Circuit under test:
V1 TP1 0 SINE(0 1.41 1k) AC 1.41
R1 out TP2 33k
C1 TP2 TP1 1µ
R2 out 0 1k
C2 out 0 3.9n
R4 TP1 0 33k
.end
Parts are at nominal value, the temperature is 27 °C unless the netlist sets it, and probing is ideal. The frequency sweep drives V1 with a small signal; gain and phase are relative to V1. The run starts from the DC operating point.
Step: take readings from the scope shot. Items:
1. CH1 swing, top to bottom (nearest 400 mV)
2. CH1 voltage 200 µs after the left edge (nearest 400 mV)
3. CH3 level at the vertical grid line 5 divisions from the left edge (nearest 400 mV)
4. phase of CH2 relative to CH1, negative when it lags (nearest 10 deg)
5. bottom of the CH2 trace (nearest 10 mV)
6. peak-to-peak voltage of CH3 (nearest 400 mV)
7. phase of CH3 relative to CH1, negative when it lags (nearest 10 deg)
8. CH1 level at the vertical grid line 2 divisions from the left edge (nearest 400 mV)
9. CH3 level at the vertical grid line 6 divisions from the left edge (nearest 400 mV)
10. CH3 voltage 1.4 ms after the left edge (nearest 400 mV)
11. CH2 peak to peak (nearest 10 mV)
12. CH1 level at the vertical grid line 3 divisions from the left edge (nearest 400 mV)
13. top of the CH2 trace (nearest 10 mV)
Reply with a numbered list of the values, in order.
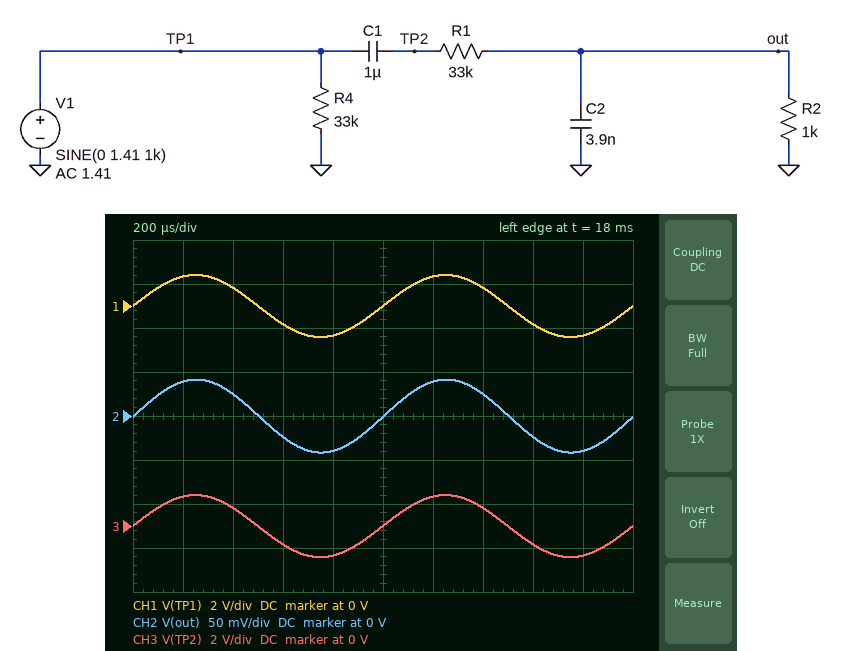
1. 2.8 V
2. 1.2 V
3. 0 V
4. 0 deg
5. -40 mV
6. 2.8 V
7. 0 deg
8. 800 mV
9. 1.2 V
10. 800 mV
11. 80 mV
12. -800 mV
13. 40 mV
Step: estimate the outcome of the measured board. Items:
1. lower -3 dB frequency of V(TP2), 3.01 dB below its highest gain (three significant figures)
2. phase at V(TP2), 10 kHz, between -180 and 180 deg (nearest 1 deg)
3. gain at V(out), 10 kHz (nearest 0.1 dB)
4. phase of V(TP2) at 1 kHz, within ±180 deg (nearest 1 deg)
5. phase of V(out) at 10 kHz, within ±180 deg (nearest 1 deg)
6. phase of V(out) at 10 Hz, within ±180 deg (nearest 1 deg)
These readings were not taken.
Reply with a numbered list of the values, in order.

1. 4.68 Hz
2. 0 deg
3. -30.9 dB
4. 0 deg
5. -13 deg
6. 25 deg
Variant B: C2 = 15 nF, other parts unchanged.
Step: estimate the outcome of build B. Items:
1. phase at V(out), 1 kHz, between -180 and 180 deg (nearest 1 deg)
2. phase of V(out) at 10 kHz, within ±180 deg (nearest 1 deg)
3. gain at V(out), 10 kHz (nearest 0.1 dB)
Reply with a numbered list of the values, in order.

1. -5 deg
2. -42 deg
3. -33.3 dB
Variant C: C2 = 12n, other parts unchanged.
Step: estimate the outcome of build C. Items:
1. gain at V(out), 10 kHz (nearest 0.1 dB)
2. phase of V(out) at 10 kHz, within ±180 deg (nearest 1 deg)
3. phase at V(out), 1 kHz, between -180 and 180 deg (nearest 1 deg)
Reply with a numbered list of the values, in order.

1. -32.5 dB
2. -36 deg
3. -4 deg
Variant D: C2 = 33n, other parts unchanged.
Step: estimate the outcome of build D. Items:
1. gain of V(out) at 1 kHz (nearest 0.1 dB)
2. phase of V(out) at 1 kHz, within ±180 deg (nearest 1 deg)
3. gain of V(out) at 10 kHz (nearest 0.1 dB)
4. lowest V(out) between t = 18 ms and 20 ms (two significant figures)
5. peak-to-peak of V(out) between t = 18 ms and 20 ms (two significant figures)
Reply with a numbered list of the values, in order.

1. -30.8 dB
2. -11 deg
3. -37.7 dB
4. -41 mV
5. 81 mV
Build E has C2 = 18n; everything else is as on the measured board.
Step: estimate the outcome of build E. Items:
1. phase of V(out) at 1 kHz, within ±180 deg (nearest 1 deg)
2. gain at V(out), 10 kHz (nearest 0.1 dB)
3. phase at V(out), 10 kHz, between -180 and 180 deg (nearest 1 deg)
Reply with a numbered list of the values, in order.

1. -6 deg
2. -34.1 dB
3. -48 deg
